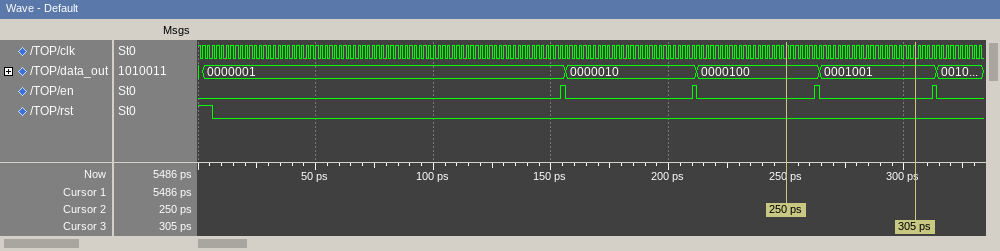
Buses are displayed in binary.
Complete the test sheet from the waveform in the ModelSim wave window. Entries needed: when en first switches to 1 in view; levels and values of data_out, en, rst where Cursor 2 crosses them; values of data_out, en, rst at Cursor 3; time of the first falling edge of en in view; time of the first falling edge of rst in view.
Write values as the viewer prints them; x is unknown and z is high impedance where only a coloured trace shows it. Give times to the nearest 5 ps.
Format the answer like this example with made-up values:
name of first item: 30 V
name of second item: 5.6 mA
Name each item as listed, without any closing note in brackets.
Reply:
when en first switches to 1 in view: 155 ps
levels and values of data_out, en, rst where Cursor 2 crosses them: data_out=0000100, en=0, rst=0
values of data_out, en, rst at Cursor 3: data_out=0001001, en=0, rst=0
time of the first falling edge of en in view: 155 ps
time of the first falling edge of rst in view: 5 ps
